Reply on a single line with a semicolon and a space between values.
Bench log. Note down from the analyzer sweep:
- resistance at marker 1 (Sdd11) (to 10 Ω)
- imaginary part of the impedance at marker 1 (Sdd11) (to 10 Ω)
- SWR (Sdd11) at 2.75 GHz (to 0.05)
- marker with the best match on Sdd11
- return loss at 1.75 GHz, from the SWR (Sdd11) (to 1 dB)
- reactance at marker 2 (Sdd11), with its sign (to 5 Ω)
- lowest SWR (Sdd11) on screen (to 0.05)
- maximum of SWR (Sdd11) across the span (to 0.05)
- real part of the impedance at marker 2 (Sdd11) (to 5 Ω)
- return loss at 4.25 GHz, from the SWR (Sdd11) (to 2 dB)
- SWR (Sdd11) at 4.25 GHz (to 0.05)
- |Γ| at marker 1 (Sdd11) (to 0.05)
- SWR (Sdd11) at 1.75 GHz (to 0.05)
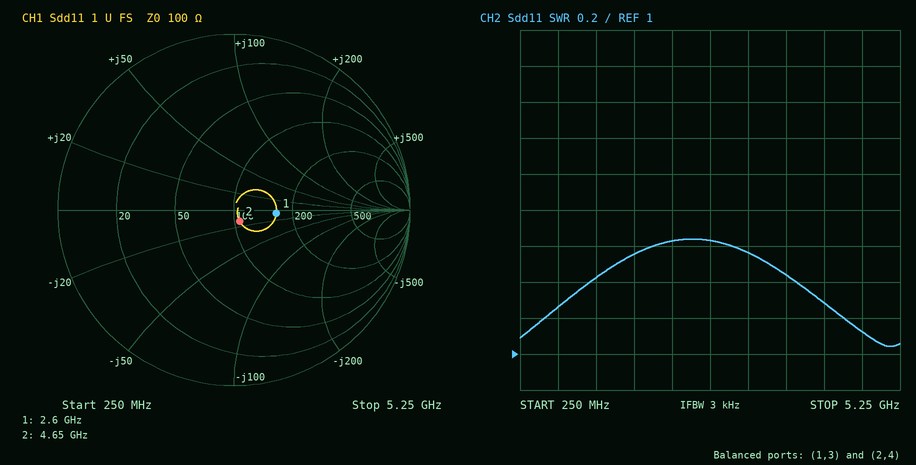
160 Ω; -10 Ω; 1.65; marker 2; 13 dB; -15 Ω; 1.05; 1.65; 105 Ω; 18 dB; 1.30; 0.25; 1.55
